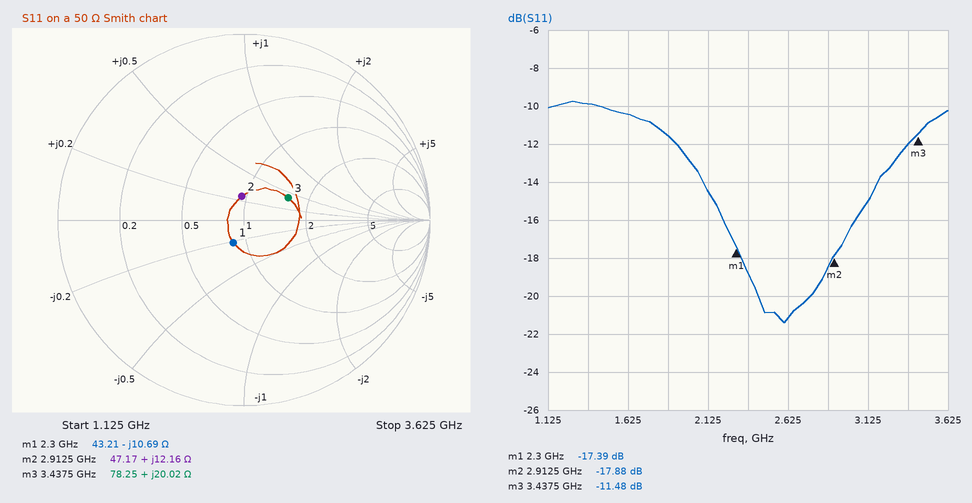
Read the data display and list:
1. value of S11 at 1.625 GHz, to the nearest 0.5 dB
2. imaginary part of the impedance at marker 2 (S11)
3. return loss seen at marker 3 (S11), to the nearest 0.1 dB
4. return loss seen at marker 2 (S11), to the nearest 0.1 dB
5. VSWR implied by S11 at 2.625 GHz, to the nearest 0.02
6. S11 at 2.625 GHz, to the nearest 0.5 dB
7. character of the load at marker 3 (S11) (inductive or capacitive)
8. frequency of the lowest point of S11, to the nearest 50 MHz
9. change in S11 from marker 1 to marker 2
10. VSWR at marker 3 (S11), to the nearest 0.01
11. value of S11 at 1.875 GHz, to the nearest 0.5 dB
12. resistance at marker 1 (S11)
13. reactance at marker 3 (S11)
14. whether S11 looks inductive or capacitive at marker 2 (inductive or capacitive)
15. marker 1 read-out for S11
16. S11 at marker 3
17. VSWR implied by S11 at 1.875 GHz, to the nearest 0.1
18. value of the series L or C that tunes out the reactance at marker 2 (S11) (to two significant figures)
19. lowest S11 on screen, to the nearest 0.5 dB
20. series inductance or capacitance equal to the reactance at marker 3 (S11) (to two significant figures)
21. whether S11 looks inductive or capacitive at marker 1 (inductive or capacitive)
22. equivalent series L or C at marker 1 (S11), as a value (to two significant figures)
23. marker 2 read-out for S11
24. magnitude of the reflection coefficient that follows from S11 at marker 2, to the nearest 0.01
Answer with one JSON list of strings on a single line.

["-10.5 dB", "+12.16 Ω", "11.5 dB", "17.9 dB", "1.20", "-21.0 dB", "inductive", "2.60 GHz", "-0.49 dB", "1.73", "-11.5 dB", "43.21 Ω", "+20.02 Ω", "inductive", "-17.39 dB", "-11.48 dB", "1.7", "4.5 pF", "-21.5 dB", "930 pH", "capacitive", "6.5 pF", "-17.88 dB", "0.13"]
